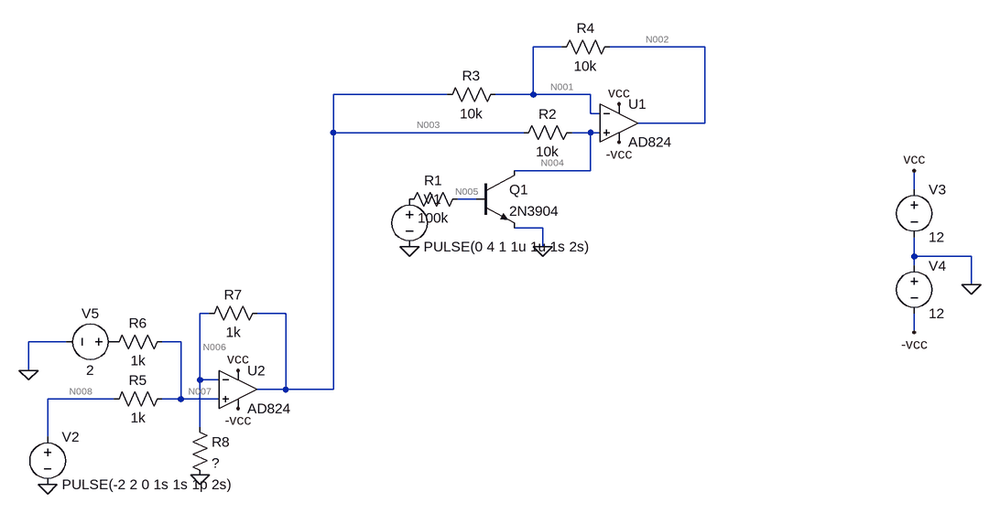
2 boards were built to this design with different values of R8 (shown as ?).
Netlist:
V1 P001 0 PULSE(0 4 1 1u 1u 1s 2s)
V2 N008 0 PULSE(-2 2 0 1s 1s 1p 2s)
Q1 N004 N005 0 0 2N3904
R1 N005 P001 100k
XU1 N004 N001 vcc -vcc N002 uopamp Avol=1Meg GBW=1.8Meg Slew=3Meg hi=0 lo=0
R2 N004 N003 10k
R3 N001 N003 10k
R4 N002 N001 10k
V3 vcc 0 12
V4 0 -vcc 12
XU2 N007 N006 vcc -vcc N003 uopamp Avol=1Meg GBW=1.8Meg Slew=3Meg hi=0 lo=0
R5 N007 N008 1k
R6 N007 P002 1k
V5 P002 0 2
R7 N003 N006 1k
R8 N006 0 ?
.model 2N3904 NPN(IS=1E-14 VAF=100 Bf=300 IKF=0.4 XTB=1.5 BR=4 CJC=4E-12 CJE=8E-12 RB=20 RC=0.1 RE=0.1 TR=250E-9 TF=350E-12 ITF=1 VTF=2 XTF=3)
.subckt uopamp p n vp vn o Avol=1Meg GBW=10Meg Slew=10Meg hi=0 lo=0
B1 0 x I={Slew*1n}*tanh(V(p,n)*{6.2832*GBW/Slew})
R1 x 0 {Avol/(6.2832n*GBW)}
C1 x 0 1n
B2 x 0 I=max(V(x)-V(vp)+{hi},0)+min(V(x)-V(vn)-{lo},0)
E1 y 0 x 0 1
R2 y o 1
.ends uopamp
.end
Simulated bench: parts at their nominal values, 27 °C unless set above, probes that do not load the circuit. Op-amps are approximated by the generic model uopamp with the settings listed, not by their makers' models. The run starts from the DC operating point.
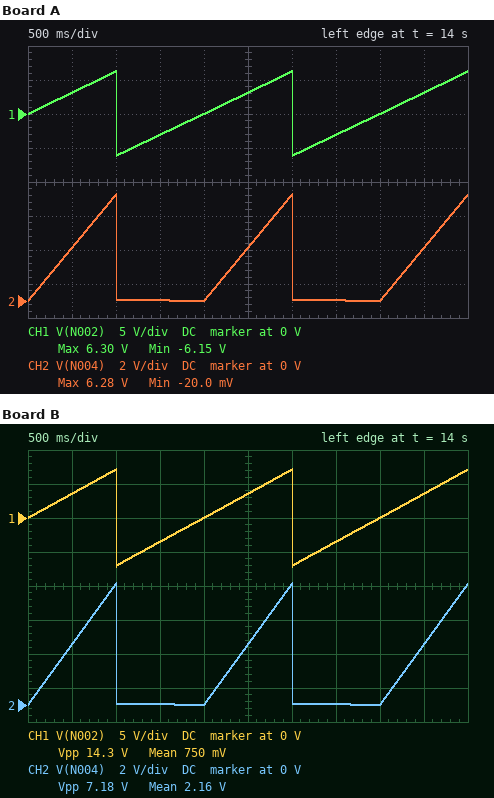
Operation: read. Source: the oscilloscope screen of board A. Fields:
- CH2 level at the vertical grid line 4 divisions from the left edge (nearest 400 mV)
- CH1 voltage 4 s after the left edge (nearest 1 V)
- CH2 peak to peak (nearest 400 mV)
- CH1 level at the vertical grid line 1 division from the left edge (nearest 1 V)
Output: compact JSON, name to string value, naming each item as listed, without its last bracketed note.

{"CH2 level at the vertical grid line 4 divisions from the left edge": "0 V", "CH1 voltage 4 s after the left edge": "0 V", "CH2 peak to peak": "6.4 V", "CH1 level at the vertical grid line 1 division from the left edge": "3 V"}
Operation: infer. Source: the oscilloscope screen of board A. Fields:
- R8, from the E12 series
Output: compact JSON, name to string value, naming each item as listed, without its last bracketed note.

{"R8, from the E12 series": "470 Ω"}
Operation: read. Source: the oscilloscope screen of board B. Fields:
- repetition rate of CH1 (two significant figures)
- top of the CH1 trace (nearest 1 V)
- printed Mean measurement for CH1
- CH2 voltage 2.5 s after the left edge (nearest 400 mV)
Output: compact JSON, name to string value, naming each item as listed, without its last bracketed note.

{"repetition rate of CH1": "500 mHz", "top of the CH1 trace": "7 V", "printed Mean measurement for CH1": "750 mV", "CH2 voltage 2.5 s after the left edge": "3.6 V"}
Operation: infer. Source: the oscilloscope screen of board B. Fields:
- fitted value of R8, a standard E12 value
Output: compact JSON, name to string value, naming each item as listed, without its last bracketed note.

{"fitted value of R8, a standard E12 value": "390 Ω"}
